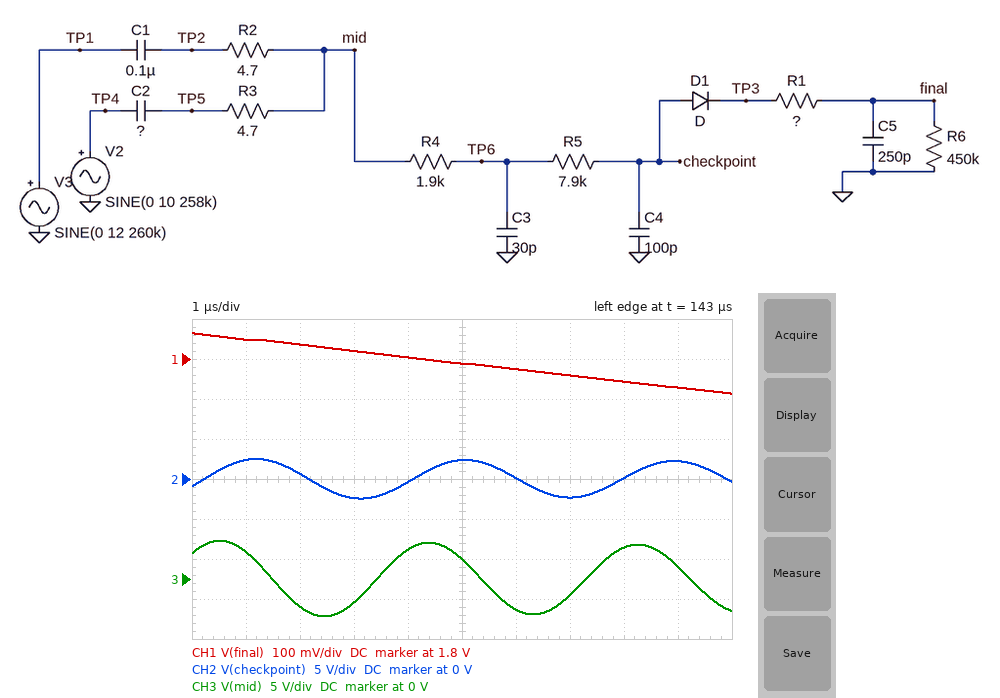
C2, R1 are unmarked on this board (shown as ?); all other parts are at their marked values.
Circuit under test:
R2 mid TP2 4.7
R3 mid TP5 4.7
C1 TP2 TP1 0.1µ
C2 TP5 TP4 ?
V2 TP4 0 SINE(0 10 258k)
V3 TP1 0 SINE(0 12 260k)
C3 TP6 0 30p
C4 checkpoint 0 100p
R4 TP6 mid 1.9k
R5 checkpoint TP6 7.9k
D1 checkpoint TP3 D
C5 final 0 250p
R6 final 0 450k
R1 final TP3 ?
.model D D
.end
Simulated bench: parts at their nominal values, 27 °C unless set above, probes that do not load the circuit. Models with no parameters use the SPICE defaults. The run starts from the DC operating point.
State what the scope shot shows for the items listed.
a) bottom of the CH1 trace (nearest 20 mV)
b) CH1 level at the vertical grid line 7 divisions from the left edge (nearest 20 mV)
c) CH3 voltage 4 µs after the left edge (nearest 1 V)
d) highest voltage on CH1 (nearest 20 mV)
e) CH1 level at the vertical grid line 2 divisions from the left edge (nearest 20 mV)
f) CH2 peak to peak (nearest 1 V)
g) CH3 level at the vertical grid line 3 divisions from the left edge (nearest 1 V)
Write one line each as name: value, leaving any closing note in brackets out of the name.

bottom of the CH1 trace: 1.72 V
CH1 level at the vertical grid line 7 divisions from the left edge: 1.76 V
CH3 voltage 4 µs after the left edge: 4 V
highest voltage on CH1: 1.86 V
CH1 level at the vertical grid line 2 divisions from the left edge: 1.84 V
CH2 peak to peak: 5 V
CH3 level at the vertical grid line 3 divisions from the left edge: -3 V
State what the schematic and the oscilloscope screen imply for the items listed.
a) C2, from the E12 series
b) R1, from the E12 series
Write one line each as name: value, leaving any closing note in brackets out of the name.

C2, from the E12 series: 270 nF
R1, from the E12 series: 39 kΩ
